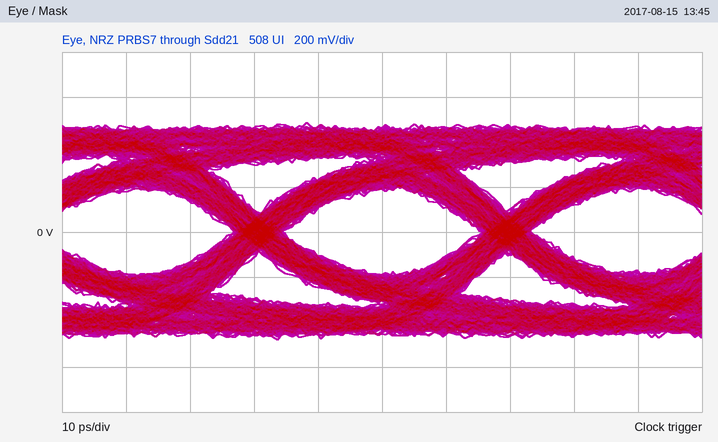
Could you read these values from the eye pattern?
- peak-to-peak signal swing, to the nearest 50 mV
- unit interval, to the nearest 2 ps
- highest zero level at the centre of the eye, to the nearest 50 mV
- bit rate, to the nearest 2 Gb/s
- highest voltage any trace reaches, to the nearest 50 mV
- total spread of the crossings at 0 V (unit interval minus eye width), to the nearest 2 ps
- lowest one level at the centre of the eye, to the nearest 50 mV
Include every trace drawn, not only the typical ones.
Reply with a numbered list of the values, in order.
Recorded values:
1. 950 mV
2. 38 ps
3. -200 mV
4. 26 Gb/s
5. 500 mV
6. 8 ps
7. 200 mV
